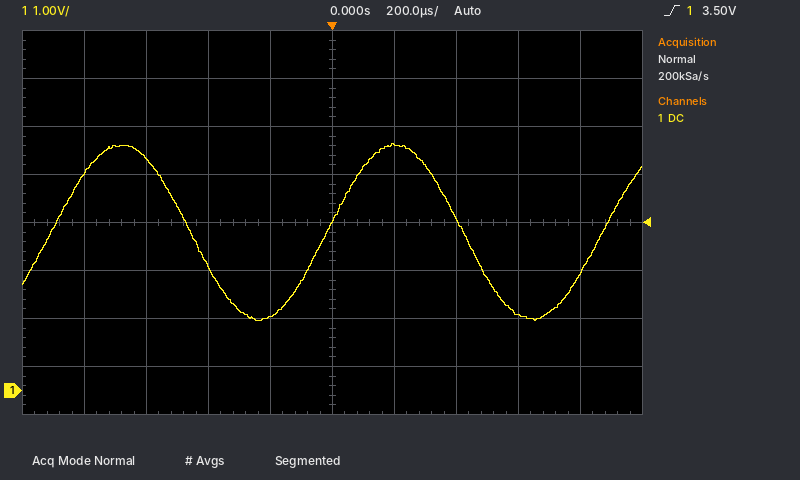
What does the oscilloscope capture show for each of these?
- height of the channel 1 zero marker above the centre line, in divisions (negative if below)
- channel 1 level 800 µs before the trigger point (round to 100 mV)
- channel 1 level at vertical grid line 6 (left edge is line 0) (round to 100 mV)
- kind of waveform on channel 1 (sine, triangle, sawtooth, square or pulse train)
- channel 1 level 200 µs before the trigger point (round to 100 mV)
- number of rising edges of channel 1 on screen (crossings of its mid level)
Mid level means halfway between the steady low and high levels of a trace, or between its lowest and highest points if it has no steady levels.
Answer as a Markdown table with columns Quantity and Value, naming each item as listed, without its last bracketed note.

| Quantity | Value |
|---|---|
| height of the channel 1 zero marker above the centre line, in divisions | -3.5 div |
| channel 1 level 800 µs before the trigger point | 4.5 V |
| channel 1 level at vertical grid line 6 (left edge is line 0) | 5.1 V |
| kind of waveform on channel 1 | sine |
| channel 1 level 200 µs before the trigger point | 1.5 V |
| number of rising edges of channel 1 on screen | 3 |
